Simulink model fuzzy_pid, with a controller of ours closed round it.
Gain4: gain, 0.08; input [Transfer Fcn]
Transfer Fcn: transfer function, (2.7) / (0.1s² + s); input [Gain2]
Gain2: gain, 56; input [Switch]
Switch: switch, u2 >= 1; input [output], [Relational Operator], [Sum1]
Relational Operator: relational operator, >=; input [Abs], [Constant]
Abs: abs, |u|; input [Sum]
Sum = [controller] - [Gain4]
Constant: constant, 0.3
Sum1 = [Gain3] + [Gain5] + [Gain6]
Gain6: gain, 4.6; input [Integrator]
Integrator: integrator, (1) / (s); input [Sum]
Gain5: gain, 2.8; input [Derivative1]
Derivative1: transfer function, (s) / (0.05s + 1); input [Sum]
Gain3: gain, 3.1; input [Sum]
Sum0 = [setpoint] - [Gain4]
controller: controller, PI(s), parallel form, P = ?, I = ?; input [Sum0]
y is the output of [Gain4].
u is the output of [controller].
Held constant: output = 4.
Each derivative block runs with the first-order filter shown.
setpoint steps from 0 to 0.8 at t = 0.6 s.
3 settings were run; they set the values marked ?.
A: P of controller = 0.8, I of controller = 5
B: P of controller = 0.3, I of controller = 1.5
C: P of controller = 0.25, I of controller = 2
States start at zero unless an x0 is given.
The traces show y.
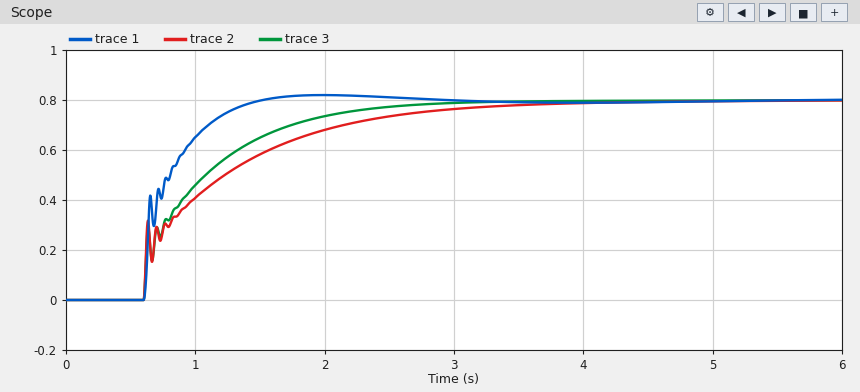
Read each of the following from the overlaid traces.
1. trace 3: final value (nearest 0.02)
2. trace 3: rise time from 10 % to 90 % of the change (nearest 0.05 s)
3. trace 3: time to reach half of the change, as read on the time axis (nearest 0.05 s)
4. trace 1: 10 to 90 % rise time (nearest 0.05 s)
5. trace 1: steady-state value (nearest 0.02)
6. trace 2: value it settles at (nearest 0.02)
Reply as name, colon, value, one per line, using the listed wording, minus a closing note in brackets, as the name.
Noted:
trace 3: final value: 0.80
trace 3: rise time from 10 % to 90 % of the change: 1.25 s
trace 3: time to reach half of the change, as read on the time axis: 0.90 s
trace 1: 10 to 90 % rise time: 0.55 s
trace 1: steady-state value: 0.80
trace 2: value it settles at: 0.80
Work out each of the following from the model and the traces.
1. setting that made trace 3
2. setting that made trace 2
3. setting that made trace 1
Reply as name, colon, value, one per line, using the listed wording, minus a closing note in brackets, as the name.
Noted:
setting that made trace 3: C
setting that made trace 2: B
setting that made trace 1: A
